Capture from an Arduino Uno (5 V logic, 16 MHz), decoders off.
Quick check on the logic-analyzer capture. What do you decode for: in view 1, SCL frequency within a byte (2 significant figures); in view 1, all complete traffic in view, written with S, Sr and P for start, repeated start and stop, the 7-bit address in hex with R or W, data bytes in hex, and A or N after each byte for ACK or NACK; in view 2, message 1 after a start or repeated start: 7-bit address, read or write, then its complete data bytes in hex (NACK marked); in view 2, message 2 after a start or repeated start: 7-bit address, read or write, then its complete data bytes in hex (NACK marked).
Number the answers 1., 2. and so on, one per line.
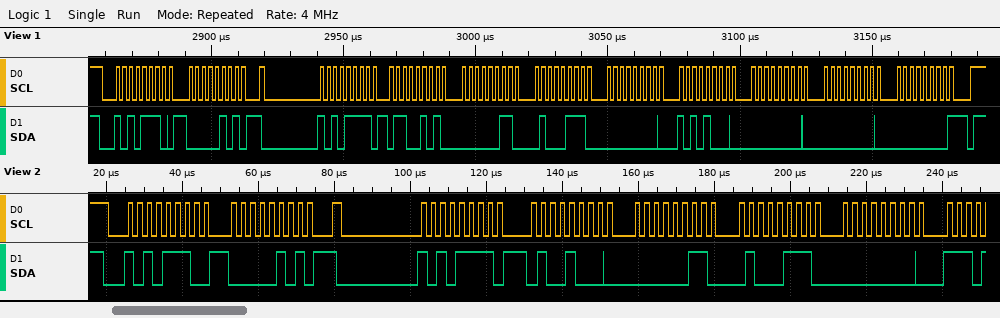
1. 400 kHz
2. S 57W A 05 A Sr 57R A 65 A 03 A 47 A 00 A A8 A 00 A 00 A 00 N P
3. 0x57 write: 05
4. 0x57 read: 48 03 47 00
